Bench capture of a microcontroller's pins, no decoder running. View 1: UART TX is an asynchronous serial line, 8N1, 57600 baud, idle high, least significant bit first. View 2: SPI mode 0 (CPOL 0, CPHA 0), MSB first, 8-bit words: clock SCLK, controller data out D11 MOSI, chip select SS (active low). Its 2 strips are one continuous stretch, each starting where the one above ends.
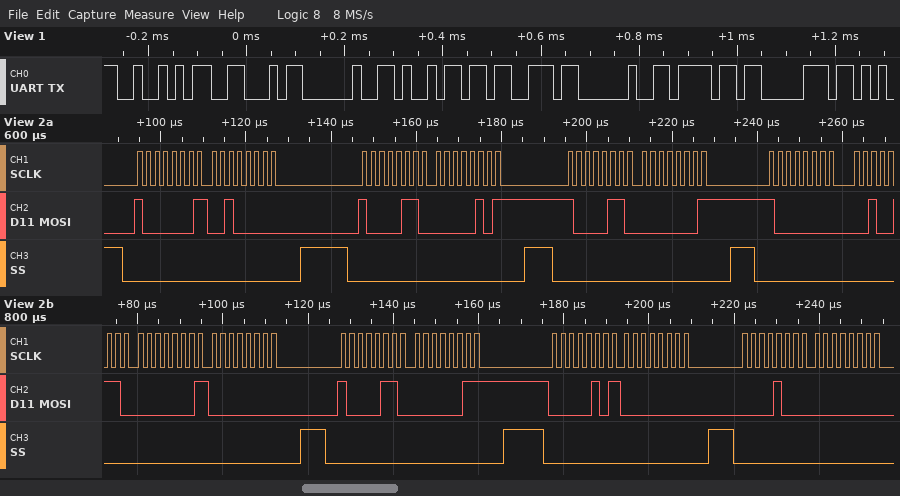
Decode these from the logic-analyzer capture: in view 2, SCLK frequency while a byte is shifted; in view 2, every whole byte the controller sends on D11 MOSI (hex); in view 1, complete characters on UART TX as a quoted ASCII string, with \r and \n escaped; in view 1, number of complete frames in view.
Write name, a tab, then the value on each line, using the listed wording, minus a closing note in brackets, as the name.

in view 2, SCLK frequency while a byte is shifted	500 kHz
in view 2, every whole byte the controller sends on D11 MOSI	81 20 86 05 86 01 80 26 01 00 86 03 05 00 08 00
in view 1, complete characters on UART TX as a quoted ASCII string, with \r and \n escaped	"RF is op"
in view 1, number of complete frames in view	8
